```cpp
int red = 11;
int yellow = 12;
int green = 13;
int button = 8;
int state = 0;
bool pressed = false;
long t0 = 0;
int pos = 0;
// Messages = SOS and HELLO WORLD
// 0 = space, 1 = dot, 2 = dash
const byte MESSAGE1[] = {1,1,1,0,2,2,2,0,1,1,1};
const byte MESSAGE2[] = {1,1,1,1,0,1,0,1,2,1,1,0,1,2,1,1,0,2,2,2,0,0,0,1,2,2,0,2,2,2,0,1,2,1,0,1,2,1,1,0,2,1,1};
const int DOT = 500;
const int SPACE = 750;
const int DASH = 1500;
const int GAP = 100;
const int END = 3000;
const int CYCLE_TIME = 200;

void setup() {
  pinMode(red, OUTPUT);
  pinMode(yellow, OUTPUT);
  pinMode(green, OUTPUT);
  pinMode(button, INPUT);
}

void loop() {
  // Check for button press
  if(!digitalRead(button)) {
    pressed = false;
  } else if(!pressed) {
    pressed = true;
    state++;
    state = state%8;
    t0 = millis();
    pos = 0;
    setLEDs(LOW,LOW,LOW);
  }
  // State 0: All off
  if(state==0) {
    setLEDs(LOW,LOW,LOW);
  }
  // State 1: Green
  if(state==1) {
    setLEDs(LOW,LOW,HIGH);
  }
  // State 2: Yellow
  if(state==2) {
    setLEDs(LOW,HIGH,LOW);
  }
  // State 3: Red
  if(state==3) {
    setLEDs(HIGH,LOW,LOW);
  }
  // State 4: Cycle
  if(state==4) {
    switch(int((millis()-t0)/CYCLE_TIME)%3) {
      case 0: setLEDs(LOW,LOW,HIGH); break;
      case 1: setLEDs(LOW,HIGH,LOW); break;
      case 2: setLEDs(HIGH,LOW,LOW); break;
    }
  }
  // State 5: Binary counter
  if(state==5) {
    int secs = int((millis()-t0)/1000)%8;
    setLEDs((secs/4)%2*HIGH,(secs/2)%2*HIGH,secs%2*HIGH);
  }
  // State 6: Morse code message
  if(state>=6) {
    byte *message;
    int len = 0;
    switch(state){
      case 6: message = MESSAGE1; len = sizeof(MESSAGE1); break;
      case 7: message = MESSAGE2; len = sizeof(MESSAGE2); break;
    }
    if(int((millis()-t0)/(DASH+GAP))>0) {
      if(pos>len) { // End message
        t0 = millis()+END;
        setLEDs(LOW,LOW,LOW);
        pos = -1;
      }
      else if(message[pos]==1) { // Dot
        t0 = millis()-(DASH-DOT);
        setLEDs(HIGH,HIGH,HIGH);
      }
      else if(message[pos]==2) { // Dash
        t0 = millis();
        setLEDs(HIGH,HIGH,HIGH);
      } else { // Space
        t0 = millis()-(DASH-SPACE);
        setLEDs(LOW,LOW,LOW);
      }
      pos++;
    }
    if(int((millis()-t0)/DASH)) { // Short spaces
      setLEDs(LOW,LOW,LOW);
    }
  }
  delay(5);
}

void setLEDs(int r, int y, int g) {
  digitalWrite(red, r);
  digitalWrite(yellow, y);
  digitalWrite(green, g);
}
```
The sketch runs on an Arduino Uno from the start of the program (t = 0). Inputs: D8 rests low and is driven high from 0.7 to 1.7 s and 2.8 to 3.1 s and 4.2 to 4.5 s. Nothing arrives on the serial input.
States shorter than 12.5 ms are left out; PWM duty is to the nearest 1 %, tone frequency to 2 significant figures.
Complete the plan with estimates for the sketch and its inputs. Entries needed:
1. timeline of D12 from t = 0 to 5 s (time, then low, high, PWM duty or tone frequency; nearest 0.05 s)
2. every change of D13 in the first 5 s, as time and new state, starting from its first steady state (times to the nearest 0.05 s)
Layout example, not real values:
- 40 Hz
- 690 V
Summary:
- 0 s low; 2.8 s high; 4.2 s low
- 0 s low; 0.7 s high; 2.8 s low
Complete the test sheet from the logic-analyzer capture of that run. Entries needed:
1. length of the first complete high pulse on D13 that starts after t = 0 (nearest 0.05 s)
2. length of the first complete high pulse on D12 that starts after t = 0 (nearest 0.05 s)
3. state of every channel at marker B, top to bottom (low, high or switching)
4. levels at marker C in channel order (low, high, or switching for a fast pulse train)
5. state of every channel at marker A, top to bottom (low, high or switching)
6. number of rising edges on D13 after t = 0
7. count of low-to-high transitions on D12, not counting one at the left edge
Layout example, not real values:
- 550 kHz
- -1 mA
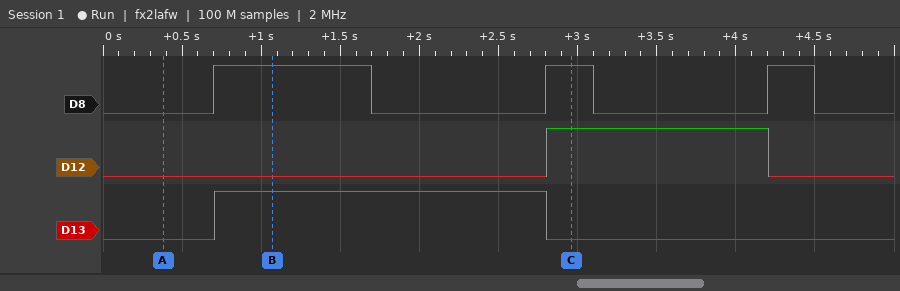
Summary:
- 2.10 s
- 1.40 s
- D8 high, D12 low, D13 high
- D8 high, D12 high, D13 low
- D8 low, D12 low, D13 low
- 1
- 1
